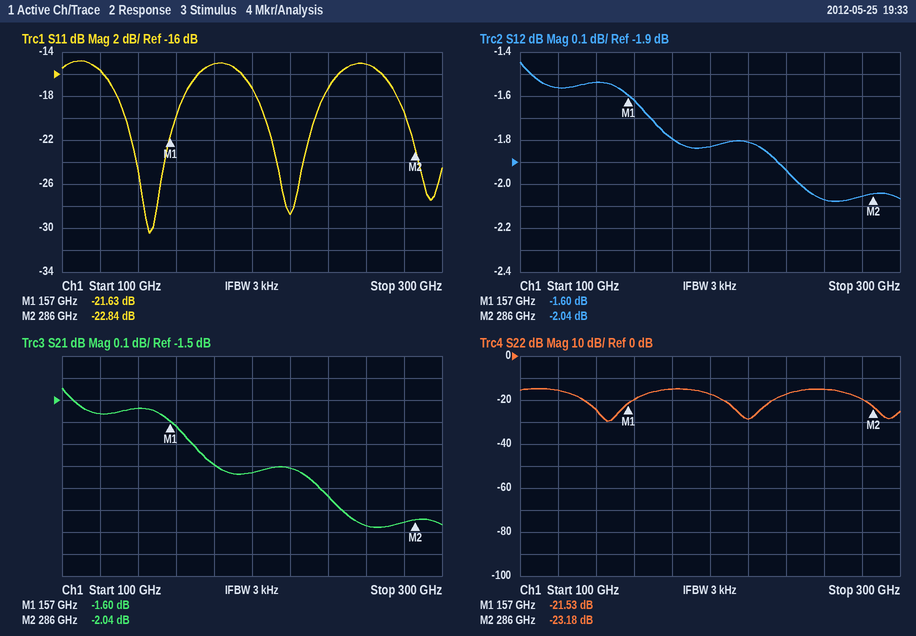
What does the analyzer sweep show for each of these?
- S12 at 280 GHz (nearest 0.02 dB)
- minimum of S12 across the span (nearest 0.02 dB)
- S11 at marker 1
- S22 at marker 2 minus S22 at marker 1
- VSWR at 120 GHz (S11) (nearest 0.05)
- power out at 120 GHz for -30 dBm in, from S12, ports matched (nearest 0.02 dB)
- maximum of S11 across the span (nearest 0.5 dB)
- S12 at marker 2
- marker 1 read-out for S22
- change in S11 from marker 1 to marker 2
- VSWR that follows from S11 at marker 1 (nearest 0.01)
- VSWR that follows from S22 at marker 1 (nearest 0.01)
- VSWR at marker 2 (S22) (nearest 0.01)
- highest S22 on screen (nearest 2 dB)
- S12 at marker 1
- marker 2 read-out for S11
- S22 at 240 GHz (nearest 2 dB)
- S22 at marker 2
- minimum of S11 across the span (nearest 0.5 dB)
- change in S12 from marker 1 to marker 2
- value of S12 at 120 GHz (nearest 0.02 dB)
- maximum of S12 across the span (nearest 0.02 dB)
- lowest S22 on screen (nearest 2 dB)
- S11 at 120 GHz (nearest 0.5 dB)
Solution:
-2.06 dB
-2.08 dB
-21.63 dB
-1.65 dB
1.40
-31.56 dBm
-15.0 dB
-2.04 dB
-21.53 dB
-1.21 dB
1.18
1.18
1.15
-14 dB
-1.60 dB
-22.84 dB
-18 dB
-23.18 dB
-30.5 dB
-0.44 dB
-1.56 dB
-1.44 dB
-30 dB
-15.5 dB
